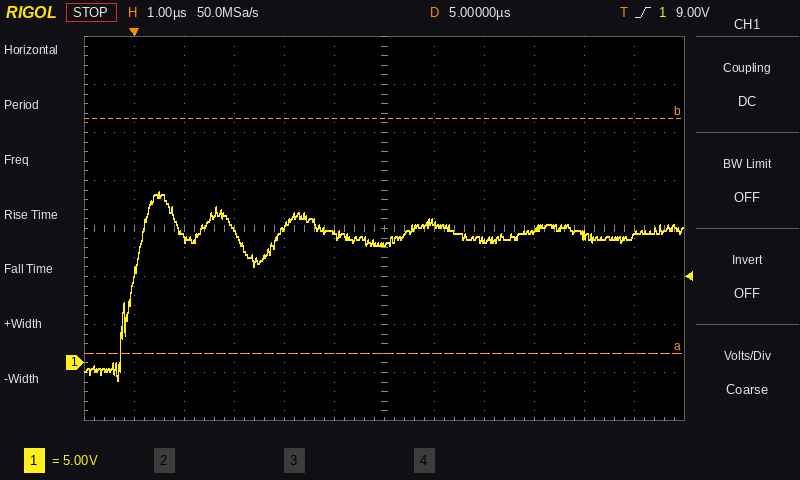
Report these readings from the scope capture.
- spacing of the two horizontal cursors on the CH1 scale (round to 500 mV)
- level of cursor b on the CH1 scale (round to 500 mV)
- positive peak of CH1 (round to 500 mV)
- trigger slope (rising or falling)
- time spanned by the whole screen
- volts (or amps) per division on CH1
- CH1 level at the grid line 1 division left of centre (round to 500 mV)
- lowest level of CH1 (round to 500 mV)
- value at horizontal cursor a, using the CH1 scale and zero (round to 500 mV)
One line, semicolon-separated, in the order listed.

24.5 V; 25.5 V; 18.0 V; rising; 12 µs; 5 V; 13.5 V; -2.0 V; 1.0 V
